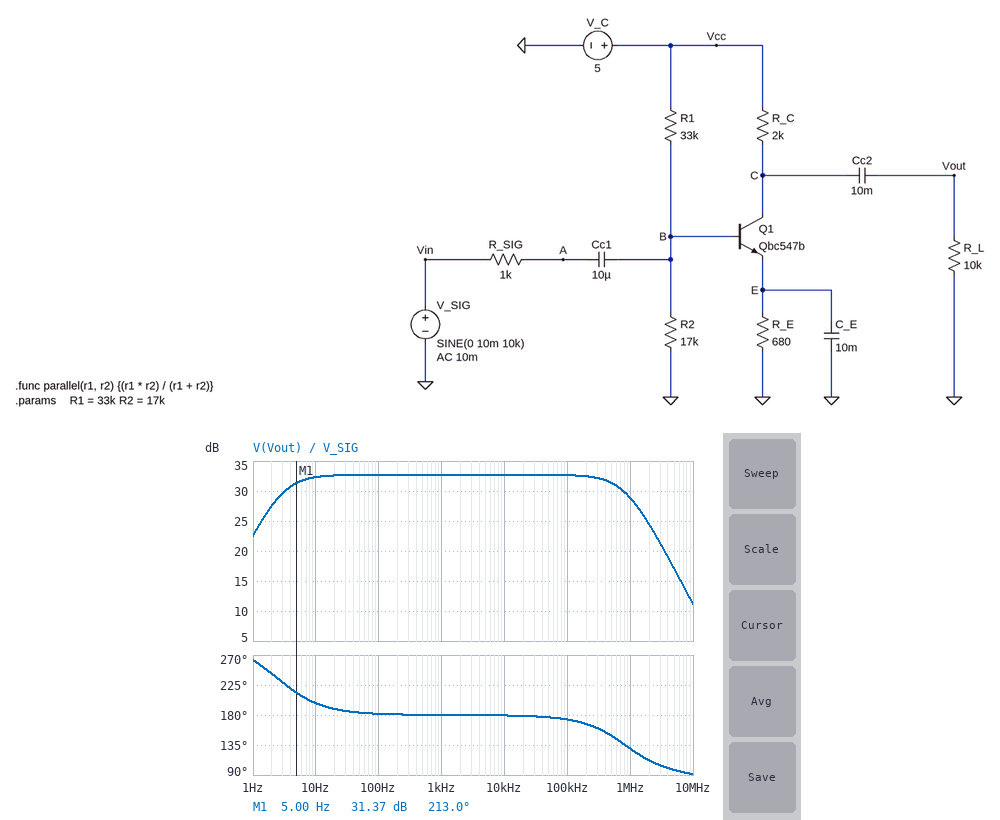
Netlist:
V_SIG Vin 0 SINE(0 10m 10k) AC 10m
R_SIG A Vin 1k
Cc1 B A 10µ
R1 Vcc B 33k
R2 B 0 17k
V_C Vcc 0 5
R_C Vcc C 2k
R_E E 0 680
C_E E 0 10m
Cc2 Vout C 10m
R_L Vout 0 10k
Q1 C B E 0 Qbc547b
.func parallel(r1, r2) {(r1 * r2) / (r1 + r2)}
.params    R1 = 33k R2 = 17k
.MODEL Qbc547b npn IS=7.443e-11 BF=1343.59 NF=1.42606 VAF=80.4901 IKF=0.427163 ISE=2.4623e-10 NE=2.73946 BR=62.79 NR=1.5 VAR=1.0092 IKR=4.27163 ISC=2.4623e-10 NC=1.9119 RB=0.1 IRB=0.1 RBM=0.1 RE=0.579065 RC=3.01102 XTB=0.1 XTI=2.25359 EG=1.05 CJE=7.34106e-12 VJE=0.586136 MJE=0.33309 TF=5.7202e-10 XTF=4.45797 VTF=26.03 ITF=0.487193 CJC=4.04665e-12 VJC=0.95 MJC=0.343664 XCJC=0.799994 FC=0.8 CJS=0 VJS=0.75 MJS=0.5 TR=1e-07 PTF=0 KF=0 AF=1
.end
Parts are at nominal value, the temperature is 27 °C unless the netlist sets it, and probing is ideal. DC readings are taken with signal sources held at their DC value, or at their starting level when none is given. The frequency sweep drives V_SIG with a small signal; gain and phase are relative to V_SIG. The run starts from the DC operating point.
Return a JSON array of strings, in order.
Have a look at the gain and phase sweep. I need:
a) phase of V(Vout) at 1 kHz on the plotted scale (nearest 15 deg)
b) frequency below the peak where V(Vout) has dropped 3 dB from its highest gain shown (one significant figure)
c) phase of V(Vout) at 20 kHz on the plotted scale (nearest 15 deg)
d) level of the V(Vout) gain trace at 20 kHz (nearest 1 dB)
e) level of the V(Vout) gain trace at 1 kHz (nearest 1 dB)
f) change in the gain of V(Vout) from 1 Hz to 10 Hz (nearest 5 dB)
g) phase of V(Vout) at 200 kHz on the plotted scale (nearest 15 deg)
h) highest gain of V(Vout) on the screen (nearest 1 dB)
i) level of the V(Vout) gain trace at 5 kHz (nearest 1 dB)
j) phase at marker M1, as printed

["180 deg", "3 Hz", "180 deg", "33 dB", "33 dB", "10 dB", "165 deg", "33 dB", "33 dB", "213.0 deg"]
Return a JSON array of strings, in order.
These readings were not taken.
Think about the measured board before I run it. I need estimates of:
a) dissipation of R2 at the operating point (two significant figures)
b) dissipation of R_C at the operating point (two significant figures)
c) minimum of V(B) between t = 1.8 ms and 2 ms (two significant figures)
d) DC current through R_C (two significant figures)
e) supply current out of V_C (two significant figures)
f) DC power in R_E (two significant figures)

["160 µW", "4.1 mW", "1.6 V", "1.4 mA", "1.5 mA", "1.4 mW"]
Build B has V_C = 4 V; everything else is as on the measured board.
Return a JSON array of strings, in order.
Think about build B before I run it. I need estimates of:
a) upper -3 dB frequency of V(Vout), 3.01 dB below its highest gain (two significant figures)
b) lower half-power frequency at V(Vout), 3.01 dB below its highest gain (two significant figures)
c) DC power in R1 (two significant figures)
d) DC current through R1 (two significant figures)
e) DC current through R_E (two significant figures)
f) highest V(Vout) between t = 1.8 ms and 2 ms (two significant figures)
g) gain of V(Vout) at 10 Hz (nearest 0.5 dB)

["1.1 MHz", "2.5 Hz", "220 µW", "81 µA", "990 µA", "290 mV", "30.0 dB"]
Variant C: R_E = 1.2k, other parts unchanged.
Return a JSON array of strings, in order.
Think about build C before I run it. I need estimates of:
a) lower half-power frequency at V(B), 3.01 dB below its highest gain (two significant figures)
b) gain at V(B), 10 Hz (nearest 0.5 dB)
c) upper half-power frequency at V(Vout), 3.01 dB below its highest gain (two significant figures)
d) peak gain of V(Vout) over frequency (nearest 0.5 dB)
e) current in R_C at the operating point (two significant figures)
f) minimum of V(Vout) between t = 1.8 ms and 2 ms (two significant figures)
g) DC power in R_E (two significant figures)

["2.3 Hz", "-1.5 dB", "1.4 MHz", "29.0 dB", "850 µA", "-310 mV", "880 µW"]
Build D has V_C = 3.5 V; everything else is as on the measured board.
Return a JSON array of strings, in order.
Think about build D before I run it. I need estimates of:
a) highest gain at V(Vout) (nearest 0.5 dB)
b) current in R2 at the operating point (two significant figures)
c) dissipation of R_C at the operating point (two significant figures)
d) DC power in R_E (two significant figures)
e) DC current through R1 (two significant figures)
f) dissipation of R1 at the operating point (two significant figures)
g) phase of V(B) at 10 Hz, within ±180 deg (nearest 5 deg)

["28.0 dB", "68 µA", "1.2 mW", "400 µW", "71 µA", "170 µW", "10 deg"]
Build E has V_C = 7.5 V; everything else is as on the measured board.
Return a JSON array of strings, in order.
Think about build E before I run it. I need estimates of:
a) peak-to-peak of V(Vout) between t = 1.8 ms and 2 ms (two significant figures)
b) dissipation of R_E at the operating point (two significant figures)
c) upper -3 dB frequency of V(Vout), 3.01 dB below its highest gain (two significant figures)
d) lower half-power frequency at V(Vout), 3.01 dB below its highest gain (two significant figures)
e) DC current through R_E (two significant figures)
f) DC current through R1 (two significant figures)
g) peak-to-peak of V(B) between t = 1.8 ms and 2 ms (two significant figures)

["1.0 V", "4.5 mW", "500 kHz", "4.2 Hz", "2.6 mA", "150 µA", "12 mV"]
